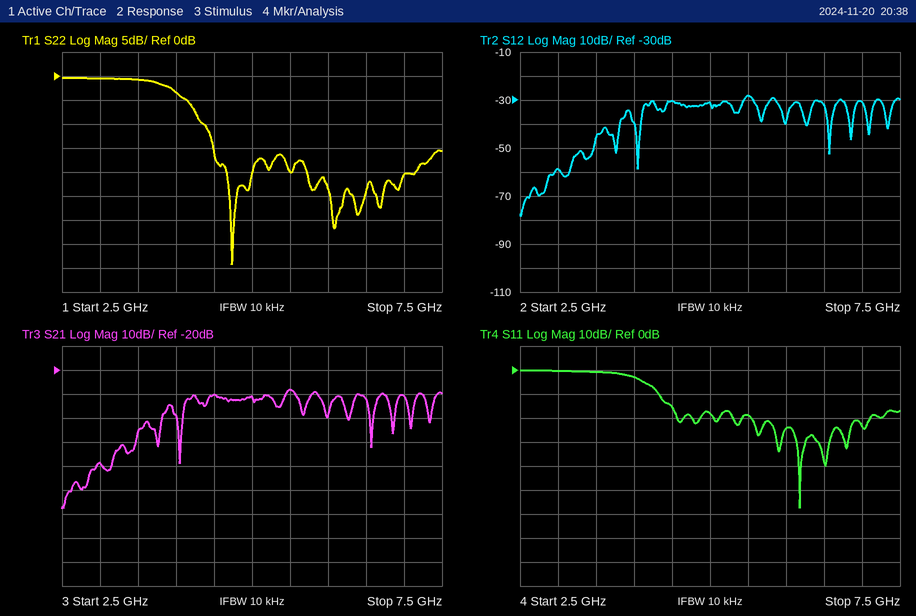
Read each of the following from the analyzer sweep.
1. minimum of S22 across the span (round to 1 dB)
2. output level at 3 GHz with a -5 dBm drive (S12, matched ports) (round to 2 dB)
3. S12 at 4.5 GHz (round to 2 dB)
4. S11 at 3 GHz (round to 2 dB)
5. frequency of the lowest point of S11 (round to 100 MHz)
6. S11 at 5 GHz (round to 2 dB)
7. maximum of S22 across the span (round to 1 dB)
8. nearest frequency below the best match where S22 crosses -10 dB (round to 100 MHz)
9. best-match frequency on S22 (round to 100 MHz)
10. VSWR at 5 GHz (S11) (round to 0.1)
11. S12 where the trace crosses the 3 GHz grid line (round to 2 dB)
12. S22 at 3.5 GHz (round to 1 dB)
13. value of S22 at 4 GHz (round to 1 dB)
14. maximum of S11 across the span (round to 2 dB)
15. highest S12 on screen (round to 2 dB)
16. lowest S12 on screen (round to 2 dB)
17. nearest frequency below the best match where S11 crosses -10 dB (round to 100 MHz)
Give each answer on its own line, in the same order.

-39 dB
-64 dBm
-30 dB
0 dB
6.2 GHz
-18 dB
0 dB
4.4 GHz
4.7 GHz
1.3
-58 dB
-1 dB
-3 dB
0 dB
-28 dB
-78 dB
4.3 GHz
